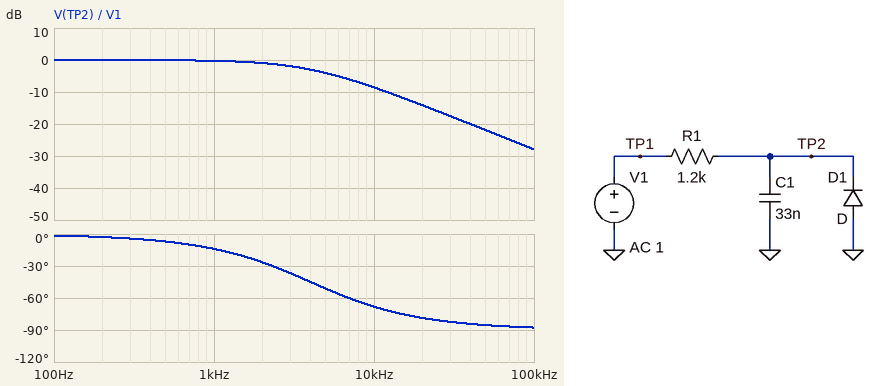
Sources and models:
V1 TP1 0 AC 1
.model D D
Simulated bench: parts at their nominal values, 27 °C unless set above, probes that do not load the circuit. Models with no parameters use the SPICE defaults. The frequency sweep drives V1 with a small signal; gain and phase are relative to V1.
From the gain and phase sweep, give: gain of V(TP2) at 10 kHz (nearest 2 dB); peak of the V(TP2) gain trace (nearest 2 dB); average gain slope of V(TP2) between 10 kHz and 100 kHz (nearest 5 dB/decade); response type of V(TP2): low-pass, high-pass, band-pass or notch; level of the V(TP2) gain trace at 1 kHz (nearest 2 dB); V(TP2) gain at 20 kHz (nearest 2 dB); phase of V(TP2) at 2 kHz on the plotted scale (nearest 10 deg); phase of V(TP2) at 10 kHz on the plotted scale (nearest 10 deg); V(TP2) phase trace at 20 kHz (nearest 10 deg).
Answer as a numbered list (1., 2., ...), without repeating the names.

1. -8 dB
2. 0 dB
3. -20 dB/decade
4. low-pass
5. 0 dB
6. -14 dB
7. -30 deg
8. -70 deg
9. -80 deg
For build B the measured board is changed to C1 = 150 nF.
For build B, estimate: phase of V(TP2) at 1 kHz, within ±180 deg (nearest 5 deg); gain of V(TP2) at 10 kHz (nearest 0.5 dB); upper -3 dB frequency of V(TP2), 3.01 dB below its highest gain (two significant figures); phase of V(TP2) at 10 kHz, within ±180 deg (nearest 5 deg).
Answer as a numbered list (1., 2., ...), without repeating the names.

1. -50 deg
2. -21.0 dB
3. 880 Hz
4. -85 deg
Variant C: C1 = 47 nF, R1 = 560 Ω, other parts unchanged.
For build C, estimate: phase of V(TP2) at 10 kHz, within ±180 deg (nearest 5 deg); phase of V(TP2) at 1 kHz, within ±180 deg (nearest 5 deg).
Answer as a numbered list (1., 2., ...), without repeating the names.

1. -60 deg
2. -10 deg
